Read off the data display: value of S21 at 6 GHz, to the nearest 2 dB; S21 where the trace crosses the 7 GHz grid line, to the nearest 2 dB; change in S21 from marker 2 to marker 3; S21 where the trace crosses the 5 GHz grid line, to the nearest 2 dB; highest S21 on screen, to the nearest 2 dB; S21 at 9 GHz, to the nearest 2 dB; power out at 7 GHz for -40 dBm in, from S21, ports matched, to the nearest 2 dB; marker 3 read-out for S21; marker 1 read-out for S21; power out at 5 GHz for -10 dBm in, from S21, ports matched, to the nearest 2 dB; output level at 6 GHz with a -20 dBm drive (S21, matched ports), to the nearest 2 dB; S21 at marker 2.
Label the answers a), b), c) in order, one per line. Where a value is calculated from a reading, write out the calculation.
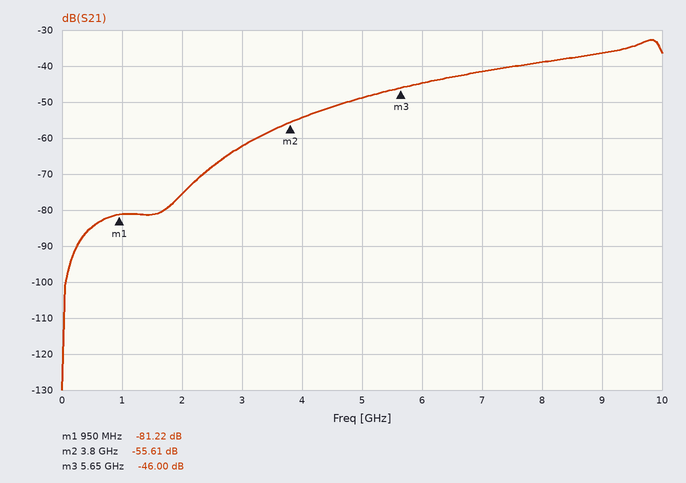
a) -44 dB
b) -42 dB
c) -46 − (-55.61) = 9.61 dB
d) -48 dB
e) -32 dB
f) -36 dB
g) -40 dBm + (-42 dB) = -82 dBm
h) -46.00 dB
i) -81.22 dB
j) -10 dBm + (-48 dB) = -58 dBm
k) -20 dBm + (-44 dB) = -64 dBm
l) -55.61 dB
